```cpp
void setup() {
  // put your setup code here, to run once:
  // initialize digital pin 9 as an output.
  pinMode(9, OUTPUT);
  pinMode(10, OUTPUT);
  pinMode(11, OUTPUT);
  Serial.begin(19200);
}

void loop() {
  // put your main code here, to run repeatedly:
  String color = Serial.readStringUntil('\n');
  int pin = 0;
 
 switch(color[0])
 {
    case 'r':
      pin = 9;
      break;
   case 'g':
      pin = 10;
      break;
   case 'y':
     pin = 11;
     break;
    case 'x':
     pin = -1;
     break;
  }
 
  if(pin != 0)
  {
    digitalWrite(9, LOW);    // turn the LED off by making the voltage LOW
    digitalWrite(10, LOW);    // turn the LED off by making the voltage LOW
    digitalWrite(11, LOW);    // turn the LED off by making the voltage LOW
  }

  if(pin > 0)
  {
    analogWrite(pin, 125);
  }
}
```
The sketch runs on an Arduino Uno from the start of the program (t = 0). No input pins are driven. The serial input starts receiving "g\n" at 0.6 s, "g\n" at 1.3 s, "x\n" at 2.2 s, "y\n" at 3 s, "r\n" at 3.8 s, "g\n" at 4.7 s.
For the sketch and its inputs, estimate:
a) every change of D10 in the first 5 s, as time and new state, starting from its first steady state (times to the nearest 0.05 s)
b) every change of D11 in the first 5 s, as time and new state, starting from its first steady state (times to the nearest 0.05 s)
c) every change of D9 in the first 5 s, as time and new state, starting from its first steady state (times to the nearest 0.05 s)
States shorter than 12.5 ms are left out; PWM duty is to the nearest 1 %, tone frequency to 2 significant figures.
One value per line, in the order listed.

0 s low; 0.6 s PWM 49 %; 2.2 s low; 4.7 s PWM 49 %
0 s low; 3 s PWM 49 %; 3.8 s low
0 s low; 3.8 s PWM 49 %; 4.7 s low
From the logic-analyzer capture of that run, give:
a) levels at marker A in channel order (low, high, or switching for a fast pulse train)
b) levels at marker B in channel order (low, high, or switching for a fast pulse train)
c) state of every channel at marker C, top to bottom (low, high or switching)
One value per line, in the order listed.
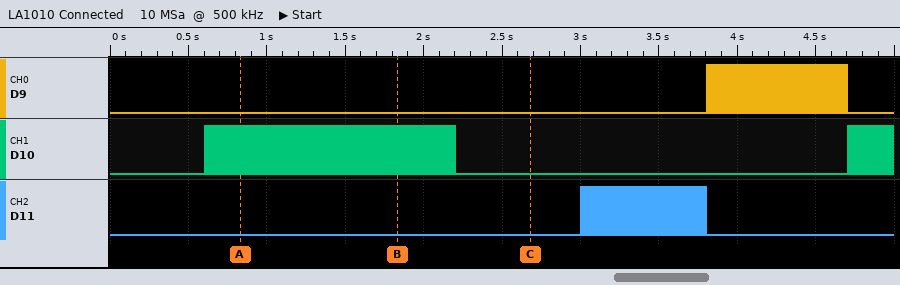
D9 low, D10 switching, D11 low
D9 low, D10 switching, D11 low
D9 low, D10 low, D11 low
